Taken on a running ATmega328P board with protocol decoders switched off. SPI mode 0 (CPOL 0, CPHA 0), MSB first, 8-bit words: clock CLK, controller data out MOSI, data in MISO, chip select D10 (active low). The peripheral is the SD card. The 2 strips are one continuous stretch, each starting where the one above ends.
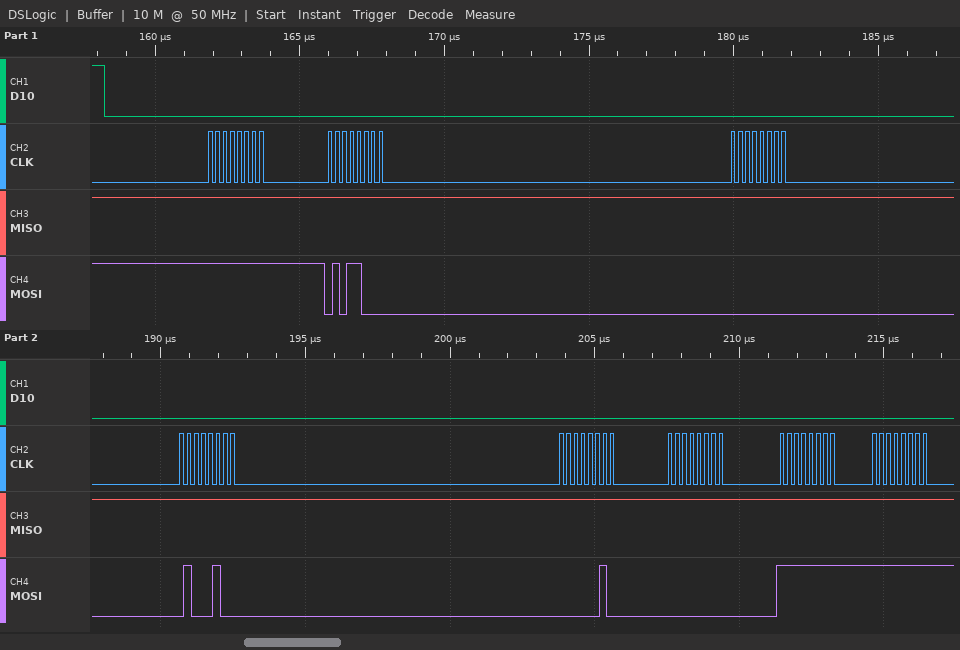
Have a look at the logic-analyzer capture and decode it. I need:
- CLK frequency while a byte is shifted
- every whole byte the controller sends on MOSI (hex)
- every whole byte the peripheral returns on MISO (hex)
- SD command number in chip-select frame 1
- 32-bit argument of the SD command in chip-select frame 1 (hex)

4 MHz
0xFF 0x58 0x00 0x44 0x02 0x00 0xFF 0xFF
0xFF 0xFF 0xFF 0xFF 0xFF 0xFF 0xFF 0xFF
CMD24
0x00440200
